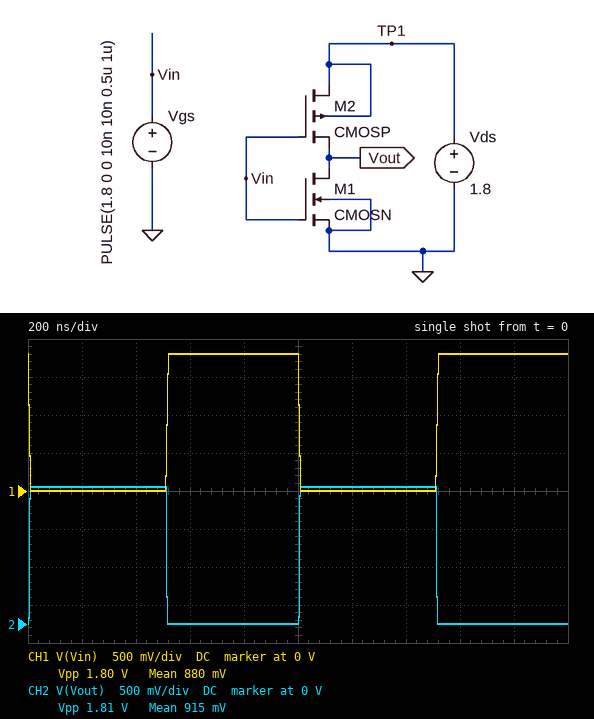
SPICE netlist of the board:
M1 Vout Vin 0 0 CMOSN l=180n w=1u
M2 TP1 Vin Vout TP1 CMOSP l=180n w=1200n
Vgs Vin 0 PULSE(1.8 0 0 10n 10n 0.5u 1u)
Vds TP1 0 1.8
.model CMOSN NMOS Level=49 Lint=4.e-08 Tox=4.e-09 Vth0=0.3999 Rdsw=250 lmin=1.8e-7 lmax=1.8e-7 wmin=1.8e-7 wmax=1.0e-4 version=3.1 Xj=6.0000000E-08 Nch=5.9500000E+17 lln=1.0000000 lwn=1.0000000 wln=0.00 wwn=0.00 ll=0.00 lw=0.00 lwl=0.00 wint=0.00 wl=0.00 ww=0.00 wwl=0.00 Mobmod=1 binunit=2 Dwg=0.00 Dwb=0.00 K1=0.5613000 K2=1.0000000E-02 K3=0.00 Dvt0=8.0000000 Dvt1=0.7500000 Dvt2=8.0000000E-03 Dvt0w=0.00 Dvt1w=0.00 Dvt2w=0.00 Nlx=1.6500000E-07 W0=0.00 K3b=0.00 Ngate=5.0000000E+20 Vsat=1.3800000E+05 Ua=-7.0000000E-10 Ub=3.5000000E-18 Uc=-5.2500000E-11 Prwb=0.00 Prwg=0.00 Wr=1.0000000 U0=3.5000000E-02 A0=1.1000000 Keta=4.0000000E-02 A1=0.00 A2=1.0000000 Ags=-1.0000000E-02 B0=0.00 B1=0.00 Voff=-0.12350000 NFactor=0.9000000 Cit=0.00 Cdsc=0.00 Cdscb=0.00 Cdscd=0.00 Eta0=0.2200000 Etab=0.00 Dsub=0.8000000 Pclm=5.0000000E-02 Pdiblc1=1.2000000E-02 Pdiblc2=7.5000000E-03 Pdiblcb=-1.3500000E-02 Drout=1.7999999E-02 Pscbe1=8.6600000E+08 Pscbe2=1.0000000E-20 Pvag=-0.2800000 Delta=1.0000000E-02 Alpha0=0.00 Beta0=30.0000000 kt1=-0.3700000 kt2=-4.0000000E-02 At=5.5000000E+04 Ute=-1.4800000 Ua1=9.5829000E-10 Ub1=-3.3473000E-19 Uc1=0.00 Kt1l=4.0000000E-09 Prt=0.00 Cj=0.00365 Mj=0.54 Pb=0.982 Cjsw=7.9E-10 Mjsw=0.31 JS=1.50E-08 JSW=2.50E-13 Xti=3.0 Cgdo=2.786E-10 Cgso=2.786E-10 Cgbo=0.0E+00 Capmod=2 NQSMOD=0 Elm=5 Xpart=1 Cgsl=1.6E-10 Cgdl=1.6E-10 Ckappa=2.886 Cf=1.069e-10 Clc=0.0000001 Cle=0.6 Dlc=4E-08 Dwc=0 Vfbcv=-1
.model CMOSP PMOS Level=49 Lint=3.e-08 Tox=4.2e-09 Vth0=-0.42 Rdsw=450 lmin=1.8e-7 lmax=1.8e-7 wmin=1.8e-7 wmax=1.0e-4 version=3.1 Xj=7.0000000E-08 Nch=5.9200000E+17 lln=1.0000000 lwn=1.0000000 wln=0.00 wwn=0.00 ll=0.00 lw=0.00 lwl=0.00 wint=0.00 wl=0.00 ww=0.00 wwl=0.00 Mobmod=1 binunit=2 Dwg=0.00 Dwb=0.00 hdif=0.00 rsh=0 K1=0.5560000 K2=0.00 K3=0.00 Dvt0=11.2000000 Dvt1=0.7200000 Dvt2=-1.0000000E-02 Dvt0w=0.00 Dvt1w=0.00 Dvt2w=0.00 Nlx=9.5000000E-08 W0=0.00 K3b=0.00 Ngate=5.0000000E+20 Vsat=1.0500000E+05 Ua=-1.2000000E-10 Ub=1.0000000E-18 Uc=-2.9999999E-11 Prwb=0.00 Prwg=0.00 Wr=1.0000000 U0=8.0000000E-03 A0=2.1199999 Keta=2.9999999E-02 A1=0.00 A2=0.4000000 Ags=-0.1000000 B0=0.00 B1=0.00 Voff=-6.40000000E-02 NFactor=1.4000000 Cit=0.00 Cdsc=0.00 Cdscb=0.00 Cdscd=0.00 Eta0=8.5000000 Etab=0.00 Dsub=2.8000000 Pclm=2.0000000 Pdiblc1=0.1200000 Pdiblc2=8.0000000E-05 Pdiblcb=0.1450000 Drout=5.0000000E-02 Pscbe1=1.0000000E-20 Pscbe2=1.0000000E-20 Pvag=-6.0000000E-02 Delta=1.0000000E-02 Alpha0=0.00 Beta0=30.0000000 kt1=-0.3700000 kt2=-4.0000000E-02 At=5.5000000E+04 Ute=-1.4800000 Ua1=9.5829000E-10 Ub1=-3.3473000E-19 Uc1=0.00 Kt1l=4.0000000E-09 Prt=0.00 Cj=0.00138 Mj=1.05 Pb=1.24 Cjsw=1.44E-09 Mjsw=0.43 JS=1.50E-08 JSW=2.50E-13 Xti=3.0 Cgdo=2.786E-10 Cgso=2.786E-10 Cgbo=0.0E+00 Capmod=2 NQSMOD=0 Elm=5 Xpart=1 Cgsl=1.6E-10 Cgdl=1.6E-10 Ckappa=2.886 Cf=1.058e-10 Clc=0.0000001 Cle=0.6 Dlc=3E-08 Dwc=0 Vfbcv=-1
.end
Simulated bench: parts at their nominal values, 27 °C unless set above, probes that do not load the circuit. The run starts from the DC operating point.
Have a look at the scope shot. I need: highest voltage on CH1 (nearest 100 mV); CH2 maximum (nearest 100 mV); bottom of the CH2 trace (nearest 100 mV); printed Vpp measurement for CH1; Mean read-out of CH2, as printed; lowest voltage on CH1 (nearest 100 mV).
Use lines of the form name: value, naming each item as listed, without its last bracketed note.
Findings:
highest voltage on CH1: 1.8 V
CH2 maximum: 1.8 V
bottom of the CH2 trace: 0 V
printed Vpp measurement for CH1: 1.80 V
Mean read-out of CH2, as printed: 915 mV
lowest voltage on CH1: 0 V
